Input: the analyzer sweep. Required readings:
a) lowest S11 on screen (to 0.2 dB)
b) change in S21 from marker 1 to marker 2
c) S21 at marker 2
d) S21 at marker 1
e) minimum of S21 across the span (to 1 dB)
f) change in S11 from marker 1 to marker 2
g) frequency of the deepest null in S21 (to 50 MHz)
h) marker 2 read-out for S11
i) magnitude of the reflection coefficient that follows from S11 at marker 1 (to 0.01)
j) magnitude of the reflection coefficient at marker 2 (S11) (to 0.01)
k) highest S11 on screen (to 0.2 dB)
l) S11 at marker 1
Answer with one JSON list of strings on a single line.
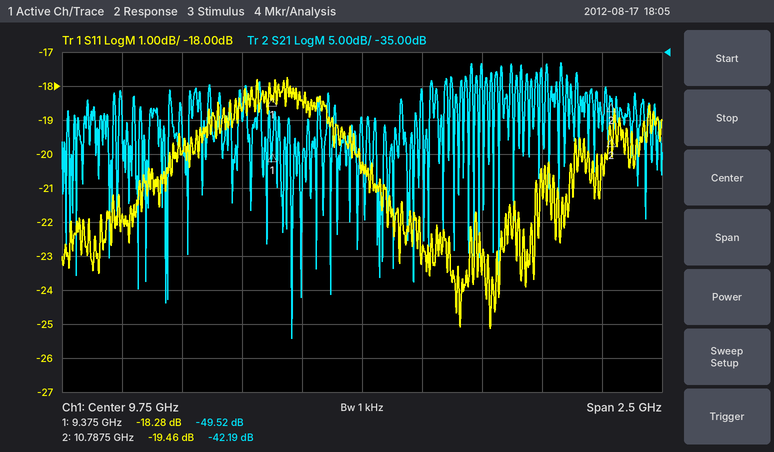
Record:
["-25.2 dB", "7.33 dB", "-42.19 dB", "-49.52 dB", "-77 dB", "-1.18 dB", "9.45 GHz", "-19.46 dB", "0.12", "0.11", "-17.8 dB", "-18.28 dB"]
